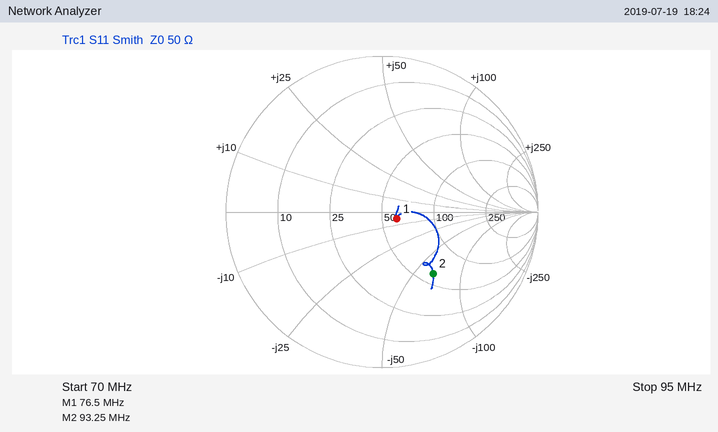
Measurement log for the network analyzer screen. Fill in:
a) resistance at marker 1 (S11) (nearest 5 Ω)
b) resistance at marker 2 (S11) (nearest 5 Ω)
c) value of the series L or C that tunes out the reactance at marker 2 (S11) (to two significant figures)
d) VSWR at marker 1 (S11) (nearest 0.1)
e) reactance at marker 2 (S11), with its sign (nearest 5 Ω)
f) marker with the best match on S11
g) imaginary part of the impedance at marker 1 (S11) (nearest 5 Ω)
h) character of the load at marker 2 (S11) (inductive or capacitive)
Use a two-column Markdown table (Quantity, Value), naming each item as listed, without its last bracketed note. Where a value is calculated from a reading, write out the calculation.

| Quantity | Value |
|---|---|
| resistance at marker 1 (S11) | 60 Ω |
| resistance at marker 2 (S11) | 60 Ω |
| value of the series L or C that tunes out the reactance at marker 2 (S11) | L = 65 Ω/(2π × 93.25 MHz) ≈ 111 nH, so 110 nH to two significant figures |
| VSWR at marker 1 (S11) | 1.2 |
| reactance at marker 2 (S11), with its sign | -65 Ω |
| marker with the best match on S11 | marker 1 |
| imaginary part of the impedance at marker 1 (S11) | -5 Ω |
| character of the load at marker 2 (S11) | capacitive |
